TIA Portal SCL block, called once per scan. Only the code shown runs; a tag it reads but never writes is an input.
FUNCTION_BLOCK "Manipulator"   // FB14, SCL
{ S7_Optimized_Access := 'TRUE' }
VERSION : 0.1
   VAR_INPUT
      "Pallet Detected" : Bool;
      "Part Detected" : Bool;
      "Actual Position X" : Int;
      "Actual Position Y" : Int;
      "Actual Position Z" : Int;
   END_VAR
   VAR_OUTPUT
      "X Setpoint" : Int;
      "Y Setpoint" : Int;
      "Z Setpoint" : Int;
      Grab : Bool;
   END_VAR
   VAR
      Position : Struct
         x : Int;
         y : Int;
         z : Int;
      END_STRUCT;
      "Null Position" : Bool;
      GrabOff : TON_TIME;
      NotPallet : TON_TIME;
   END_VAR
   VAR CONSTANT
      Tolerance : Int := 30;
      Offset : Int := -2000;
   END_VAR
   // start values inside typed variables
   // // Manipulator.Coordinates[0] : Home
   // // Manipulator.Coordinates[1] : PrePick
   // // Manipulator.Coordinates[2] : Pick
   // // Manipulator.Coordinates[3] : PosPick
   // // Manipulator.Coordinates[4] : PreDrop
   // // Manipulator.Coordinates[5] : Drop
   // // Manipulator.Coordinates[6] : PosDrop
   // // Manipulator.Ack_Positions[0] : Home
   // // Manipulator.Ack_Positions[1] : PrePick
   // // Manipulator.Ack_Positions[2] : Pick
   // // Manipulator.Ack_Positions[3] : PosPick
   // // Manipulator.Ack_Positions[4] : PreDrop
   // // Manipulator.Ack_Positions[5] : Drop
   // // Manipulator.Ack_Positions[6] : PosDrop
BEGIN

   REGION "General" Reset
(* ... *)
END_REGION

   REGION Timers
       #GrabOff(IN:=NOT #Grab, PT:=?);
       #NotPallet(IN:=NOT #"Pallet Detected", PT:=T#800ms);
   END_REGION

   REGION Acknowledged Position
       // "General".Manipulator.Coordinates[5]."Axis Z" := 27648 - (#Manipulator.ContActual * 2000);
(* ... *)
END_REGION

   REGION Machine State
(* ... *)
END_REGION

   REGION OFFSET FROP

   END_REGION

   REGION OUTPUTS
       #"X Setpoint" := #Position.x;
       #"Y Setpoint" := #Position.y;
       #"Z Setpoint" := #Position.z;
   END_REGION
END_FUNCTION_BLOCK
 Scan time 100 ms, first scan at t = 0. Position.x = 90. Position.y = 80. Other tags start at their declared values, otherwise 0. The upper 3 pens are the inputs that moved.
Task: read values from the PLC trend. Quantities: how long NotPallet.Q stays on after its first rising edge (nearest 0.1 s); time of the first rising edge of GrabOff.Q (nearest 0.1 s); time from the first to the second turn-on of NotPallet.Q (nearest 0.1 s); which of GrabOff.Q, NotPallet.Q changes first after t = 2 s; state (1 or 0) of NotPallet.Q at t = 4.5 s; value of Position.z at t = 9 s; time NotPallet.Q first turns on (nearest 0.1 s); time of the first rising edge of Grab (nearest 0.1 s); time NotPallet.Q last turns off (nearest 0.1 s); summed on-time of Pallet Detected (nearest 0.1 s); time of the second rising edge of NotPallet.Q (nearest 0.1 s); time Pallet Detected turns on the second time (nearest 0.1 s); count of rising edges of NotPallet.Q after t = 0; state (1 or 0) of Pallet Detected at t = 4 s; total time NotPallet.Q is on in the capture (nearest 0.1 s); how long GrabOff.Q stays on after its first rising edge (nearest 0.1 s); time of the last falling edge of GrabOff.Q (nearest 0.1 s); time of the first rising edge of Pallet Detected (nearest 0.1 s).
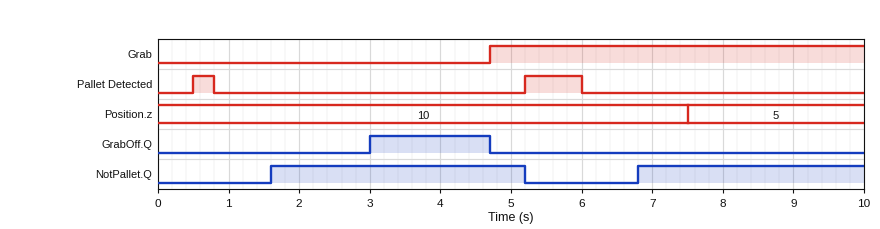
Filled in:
3.6 s
3.0 s
5.2 s
GrabOff.Q
1
5
1.6 s
4.7 s
5.2 s
1.1 s
6.8 s
5.2 s
2
0
6.8 s
1.7 s
4.7 s
0.5 s
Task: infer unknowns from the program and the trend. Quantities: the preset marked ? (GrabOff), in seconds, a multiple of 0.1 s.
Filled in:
3.0 s
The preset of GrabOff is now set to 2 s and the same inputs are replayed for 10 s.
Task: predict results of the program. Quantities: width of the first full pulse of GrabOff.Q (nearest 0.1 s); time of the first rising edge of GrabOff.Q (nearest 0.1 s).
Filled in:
2.7 s
2.0 s
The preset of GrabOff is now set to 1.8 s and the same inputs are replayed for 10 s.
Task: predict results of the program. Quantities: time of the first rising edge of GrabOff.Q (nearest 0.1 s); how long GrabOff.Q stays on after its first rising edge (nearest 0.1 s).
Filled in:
1.8 s
2.9 s
